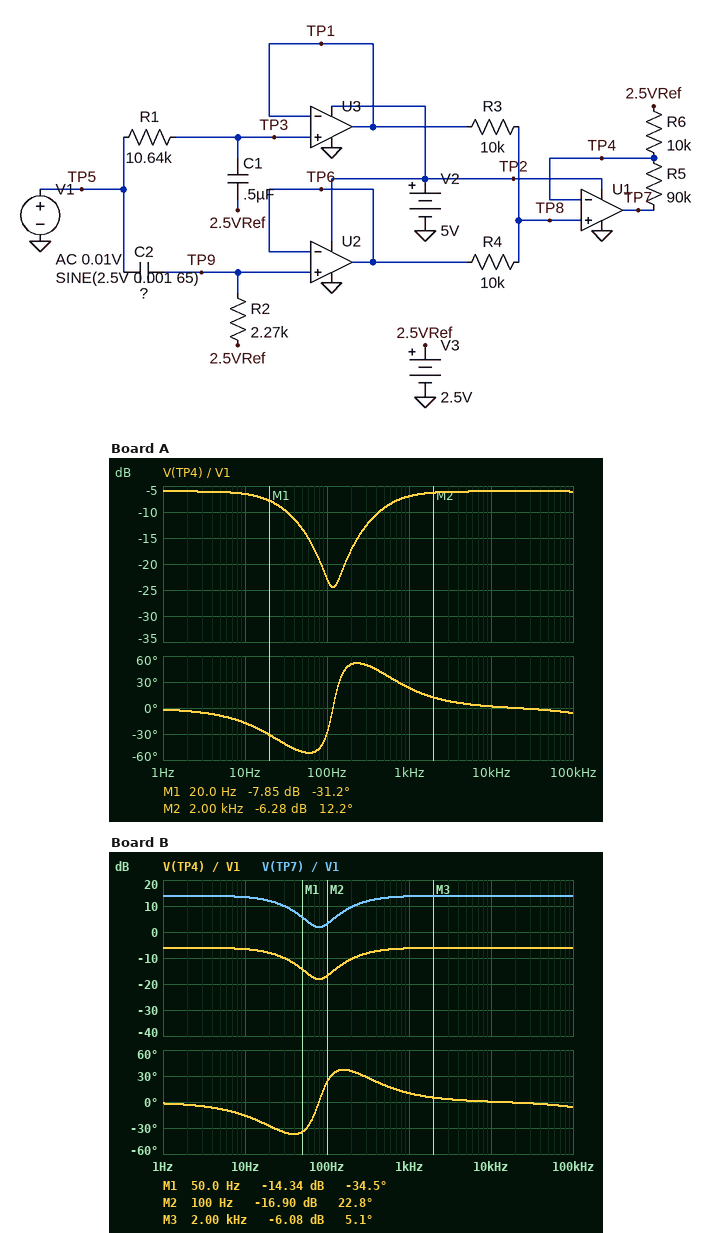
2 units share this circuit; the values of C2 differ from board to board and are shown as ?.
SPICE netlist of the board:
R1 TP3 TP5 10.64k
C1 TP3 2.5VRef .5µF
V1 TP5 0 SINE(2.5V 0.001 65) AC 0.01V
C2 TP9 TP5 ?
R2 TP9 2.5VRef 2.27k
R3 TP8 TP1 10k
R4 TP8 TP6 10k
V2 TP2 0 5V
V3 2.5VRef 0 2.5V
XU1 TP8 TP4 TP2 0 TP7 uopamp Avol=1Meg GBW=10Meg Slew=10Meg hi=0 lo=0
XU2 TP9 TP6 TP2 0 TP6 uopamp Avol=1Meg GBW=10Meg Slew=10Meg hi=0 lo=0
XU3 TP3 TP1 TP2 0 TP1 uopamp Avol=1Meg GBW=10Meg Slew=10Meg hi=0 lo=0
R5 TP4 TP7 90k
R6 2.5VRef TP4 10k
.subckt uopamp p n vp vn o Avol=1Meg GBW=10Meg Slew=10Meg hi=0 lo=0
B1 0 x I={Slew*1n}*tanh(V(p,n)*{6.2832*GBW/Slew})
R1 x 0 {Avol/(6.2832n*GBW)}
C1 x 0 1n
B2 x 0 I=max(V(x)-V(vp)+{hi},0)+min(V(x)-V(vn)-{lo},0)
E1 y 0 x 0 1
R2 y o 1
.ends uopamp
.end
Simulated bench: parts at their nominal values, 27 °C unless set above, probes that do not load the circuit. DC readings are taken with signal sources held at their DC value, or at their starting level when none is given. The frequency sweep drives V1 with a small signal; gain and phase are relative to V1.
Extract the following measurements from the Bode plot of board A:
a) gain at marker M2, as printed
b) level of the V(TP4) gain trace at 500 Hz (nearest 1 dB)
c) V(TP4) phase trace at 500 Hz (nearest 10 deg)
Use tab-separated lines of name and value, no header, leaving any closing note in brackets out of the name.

gain at marker M2, as printed	-6.28 dB
level of the V(TP4) gain trace at 500 Hz	-9 dB
V(TP4) phase trace at 500 Hz	40 deg
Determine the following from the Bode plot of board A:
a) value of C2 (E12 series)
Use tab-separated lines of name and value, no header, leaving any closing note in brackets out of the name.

value of C2	150 nF
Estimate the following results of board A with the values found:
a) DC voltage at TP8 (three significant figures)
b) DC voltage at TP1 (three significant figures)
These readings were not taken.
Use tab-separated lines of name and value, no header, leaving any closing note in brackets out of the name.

DC voltage at TP8	2.50 V
DC voltage at TP1	2.50 V
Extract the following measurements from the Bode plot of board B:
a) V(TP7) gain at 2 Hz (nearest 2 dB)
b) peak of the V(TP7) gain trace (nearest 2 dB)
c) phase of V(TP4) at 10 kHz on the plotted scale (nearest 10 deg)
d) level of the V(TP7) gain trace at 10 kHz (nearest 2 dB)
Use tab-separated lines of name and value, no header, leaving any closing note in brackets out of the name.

V(TP7) gain at 2 Hz	14 dB
peak of the V(TP7) gain trace	14 dB
phase of V(TP4) at 10 kHz on the plotted scale	0 deg
level of the V(TP7) gain trace at 10 kHz	14 dB
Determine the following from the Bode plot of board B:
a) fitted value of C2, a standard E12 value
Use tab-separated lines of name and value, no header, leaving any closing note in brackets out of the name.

fitted value of C2, a standard E12 value	330 nF
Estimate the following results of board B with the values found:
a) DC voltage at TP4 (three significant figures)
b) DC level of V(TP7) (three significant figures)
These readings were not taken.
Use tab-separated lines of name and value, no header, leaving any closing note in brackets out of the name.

DC voltage at TP4	2.50 V
DC level of V(TP7)	2.50 V
